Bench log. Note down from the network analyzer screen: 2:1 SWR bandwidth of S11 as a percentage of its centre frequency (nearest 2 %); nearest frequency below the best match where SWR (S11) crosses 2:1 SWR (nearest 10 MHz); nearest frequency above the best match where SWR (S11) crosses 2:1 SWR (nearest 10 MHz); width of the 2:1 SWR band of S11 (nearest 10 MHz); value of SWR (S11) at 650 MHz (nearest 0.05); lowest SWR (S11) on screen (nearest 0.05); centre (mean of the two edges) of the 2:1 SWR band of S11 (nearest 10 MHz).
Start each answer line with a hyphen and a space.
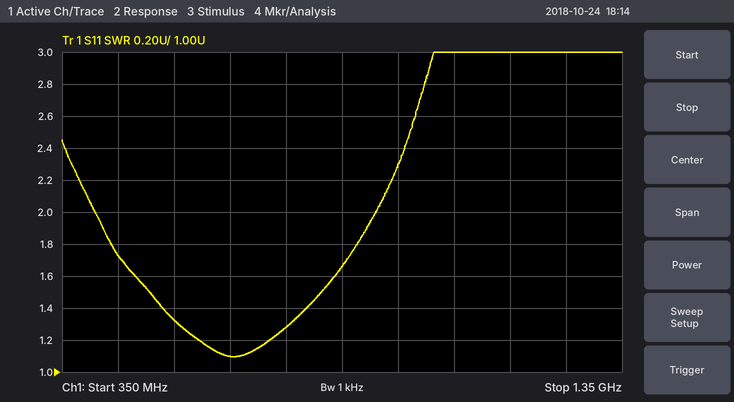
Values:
- 76 %
- 410 MHz
- 910 MHz
- 500 MHz
- 1.10
- 1.10
- 660 MHz
